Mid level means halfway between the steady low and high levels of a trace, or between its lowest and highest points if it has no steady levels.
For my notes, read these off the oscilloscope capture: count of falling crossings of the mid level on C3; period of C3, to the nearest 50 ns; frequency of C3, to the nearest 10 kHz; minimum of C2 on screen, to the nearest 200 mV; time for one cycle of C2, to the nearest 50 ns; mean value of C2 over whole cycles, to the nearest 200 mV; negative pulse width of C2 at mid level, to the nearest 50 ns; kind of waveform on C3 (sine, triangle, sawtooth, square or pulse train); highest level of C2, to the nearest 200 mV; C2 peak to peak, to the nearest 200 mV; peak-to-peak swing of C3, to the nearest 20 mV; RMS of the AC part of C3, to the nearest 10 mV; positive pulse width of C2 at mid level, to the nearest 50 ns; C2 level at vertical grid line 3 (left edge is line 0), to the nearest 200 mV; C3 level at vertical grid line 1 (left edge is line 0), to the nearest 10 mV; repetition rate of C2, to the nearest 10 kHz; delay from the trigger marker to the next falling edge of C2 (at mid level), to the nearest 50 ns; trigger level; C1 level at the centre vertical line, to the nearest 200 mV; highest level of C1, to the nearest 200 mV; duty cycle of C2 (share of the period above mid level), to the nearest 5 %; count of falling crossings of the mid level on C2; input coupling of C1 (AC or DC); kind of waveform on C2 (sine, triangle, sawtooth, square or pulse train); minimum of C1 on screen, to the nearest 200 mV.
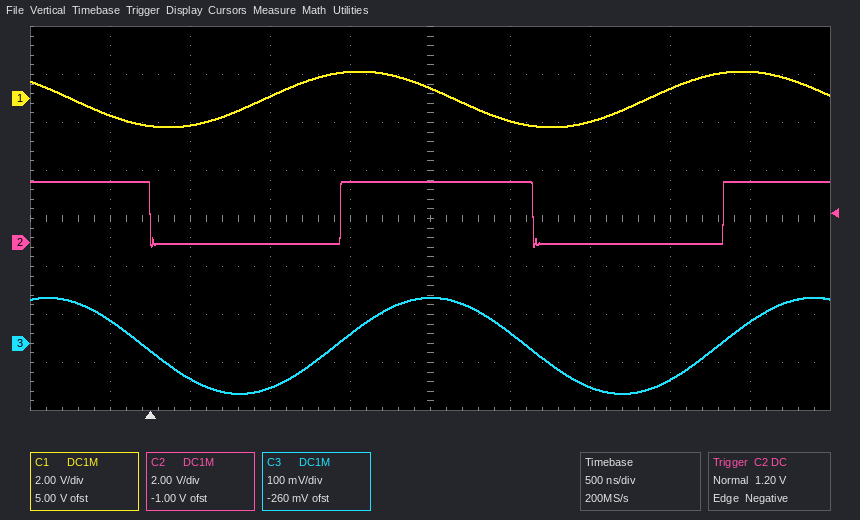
2
2.40 µs
420 kHz
-200 mV
2.40 µs
1.2 V
1.20 µs
sine
2.6 V
2.8 V
200 mV
70 mV
1.20 µs
0.0 V
50 mV
420 kHz
2.40 µs
1.20 V
400 mV
1.2 V
50 %
2
DC
square
-1.2 V
